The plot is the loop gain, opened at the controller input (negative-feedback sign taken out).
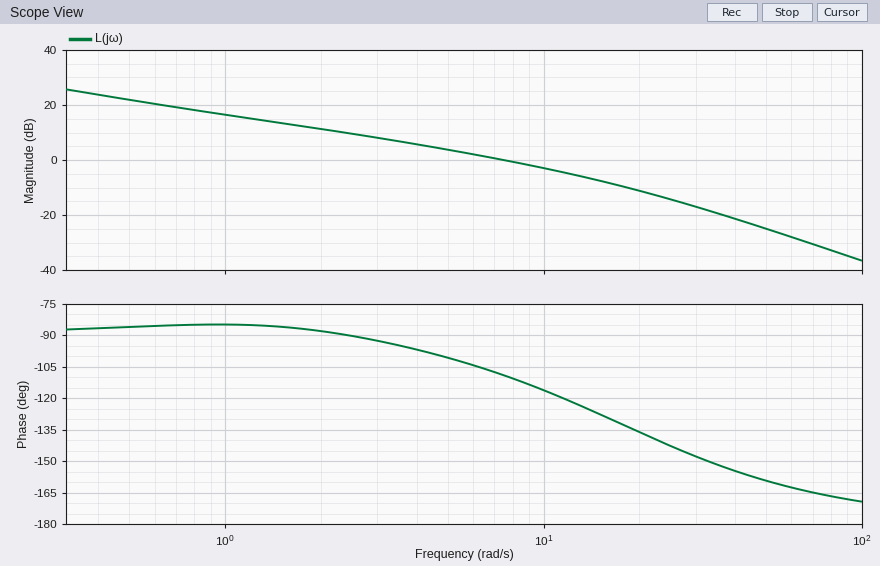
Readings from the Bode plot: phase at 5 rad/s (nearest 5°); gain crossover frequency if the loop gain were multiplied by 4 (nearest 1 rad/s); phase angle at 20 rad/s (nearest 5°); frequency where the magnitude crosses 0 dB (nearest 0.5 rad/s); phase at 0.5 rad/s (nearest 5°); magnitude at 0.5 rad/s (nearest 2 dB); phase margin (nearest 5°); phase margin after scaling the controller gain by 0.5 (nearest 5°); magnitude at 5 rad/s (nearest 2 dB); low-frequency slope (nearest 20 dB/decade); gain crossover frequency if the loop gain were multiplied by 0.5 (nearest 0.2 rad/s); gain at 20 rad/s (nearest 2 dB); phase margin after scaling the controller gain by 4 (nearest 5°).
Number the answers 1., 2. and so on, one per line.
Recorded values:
1. -100°
2. 21 rad/s
3. -135°
4. 7.5 rad/s
5. -85°
6. 22 dB
7. 70°
8. 85°
9. 4 dB
10. -20 dB/decade
11. 3.8 rad/s
12. -12 dB
13. 40°
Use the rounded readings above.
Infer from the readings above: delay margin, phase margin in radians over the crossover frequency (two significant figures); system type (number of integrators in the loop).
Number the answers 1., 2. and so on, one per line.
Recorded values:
1. 0.16 s
2. 1
